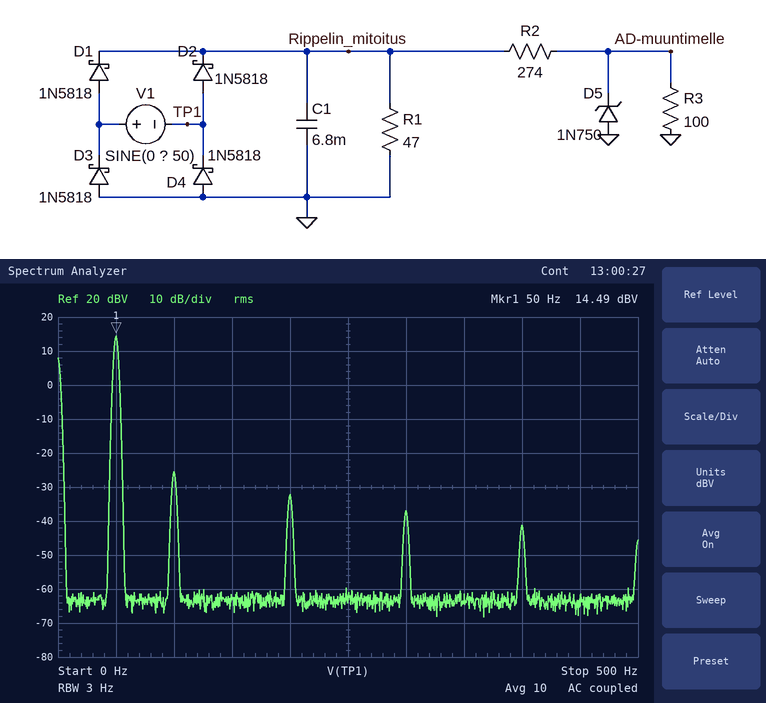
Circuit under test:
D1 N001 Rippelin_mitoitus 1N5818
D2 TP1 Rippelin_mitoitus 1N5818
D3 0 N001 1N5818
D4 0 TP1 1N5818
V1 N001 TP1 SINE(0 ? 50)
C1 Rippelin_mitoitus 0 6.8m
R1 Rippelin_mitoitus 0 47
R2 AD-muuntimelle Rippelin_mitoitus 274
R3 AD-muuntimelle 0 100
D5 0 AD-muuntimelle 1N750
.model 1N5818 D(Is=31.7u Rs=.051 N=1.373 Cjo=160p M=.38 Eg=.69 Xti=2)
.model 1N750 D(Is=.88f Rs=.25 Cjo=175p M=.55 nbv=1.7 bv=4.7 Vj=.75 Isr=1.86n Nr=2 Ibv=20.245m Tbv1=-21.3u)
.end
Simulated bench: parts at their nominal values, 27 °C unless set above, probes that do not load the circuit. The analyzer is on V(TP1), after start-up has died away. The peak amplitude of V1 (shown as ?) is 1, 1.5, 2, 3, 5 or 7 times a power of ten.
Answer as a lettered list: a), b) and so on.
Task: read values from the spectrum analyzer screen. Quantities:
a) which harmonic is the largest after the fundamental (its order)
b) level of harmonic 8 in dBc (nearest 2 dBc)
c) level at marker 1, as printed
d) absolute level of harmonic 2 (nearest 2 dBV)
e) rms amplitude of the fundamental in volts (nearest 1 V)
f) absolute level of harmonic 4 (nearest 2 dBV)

a) 2
b) -56 dBc
c) 14.49 dBV
d) -26 dBV
e) 5 V
f) -32 dBV
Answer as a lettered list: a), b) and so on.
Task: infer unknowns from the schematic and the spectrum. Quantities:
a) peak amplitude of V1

a) 15 V
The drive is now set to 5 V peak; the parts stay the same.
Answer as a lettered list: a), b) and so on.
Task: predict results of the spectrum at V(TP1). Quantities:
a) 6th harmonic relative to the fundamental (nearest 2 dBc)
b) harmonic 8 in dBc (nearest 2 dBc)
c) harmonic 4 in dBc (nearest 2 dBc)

a) -54 dBc
b) -58 dBc
c) -48 dBc
